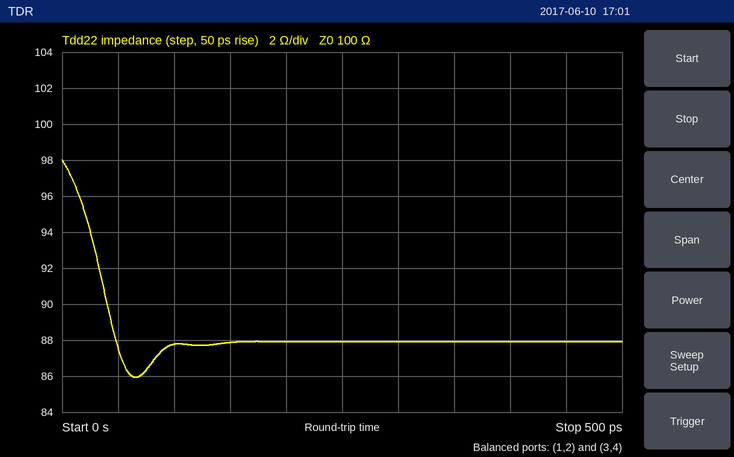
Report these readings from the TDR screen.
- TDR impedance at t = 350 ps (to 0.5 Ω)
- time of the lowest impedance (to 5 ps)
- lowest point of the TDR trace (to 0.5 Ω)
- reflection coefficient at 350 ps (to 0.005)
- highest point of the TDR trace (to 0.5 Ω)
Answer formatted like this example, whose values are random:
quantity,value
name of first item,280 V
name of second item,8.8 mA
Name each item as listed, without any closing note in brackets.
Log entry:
quantity,value
TDR impedance at t = 350 ps,88.0 Ω
time of the lowest impedance,65 ps
lowest point of the TDR trace,86.0 Ω
reflection coefficient at 350 ps,-0.065
highest point of the TDR trace,98.0 Ω
